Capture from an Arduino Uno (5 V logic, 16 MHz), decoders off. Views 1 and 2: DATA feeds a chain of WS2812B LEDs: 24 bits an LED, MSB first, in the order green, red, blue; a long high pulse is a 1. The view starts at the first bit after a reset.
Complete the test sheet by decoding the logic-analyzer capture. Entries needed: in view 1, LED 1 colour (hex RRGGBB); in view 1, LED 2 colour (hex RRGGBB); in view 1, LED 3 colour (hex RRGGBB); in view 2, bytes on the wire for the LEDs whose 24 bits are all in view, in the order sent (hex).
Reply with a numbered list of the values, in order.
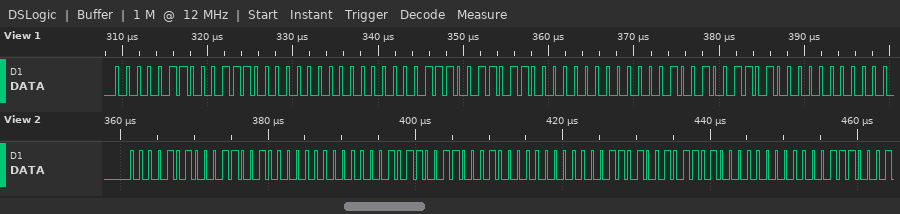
1. #380600
2. #360700
3. #340900
4. 0A 32 00 0B 31 00 0D 2D 00
